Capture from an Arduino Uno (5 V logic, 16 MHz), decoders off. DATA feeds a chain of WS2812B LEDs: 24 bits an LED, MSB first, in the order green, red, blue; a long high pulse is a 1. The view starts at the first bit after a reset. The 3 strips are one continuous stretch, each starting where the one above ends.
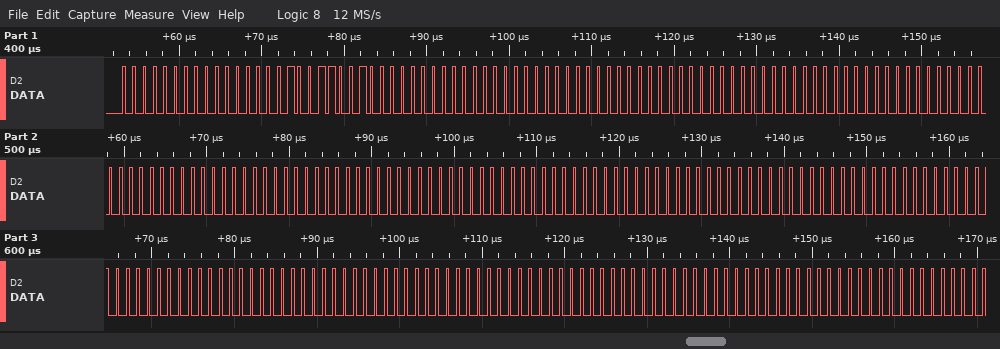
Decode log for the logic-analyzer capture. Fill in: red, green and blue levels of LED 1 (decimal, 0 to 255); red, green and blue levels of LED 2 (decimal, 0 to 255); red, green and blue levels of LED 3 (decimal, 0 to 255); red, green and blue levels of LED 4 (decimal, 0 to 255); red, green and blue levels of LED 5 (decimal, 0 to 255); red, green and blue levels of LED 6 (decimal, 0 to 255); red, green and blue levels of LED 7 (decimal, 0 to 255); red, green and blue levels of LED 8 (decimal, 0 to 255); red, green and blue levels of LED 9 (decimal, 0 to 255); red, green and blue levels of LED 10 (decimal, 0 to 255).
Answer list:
0, 0, 153
0, 0, 0
0, 0, 0
0, 0, 0
0, 0, 0
0, 0, 0
0, 0, 0
0, 0, 0
0, 0, 0
0, 0, 0
